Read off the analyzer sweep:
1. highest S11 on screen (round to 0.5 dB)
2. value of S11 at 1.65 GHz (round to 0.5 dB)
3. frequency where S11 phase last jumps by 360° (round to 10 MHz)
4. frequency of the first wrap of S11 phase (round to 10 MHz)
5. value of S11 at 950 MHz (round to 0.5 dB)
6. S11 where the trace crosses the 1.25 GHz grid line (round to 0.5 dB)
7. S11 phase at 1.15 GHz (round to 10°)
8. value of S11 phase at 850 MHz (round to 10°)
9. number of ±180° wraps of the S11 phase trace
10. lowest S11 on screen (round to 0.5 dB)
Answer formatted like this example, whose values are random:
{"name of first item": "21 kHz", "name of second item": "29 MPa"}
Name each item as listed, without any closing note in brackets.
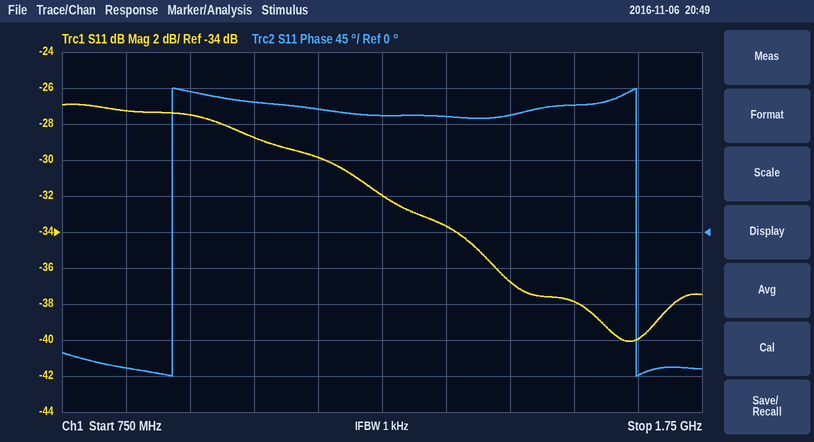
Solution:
{"highest S11 on screen": "-27.0 dB", "value of S11 at 1.65 GHz": "-40.0 dB", "frequency where S11 phase last jumps by 360°": "1.65 GHz", "frequency of the first wrap of S11 phase": "920 MHz", "value of S11 at 950 MHz": "-27.5 dB", "S11 where the trace crosses the 1.25 GHz grid line": "-32.0 dB", "S11 phase at 1.15 GHz": "150°", "value of S11 phase at 850 MHz": "-170°", "number of ±180° wraps of the S11 phase trace": "2", "lowest S11 on screen": "-40.0 dB"}
